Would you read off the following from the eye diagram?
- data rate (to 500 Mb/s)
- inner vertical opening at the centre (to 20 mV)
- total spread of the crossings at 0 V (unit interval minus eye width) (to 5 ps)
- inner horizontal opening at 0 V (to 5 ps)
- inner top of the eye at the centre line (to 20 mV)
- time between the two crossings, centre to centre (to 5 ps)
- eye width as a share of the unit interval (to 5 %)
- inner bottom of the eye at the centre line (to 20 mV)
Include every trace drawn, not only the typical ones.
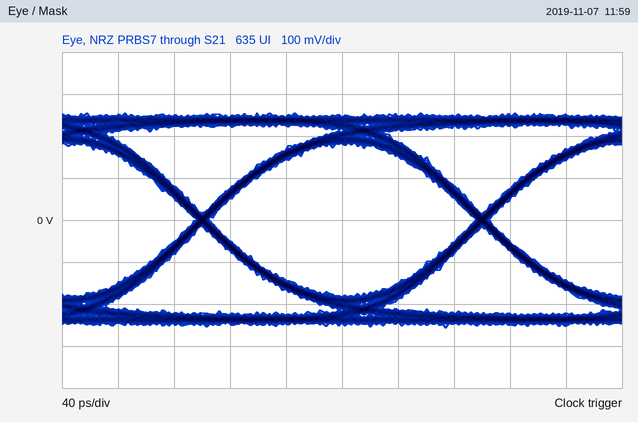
5.0 Gb/s
360 mV
10 ps
190 ps
180 mV
200 ps
95 %
-180 mV
